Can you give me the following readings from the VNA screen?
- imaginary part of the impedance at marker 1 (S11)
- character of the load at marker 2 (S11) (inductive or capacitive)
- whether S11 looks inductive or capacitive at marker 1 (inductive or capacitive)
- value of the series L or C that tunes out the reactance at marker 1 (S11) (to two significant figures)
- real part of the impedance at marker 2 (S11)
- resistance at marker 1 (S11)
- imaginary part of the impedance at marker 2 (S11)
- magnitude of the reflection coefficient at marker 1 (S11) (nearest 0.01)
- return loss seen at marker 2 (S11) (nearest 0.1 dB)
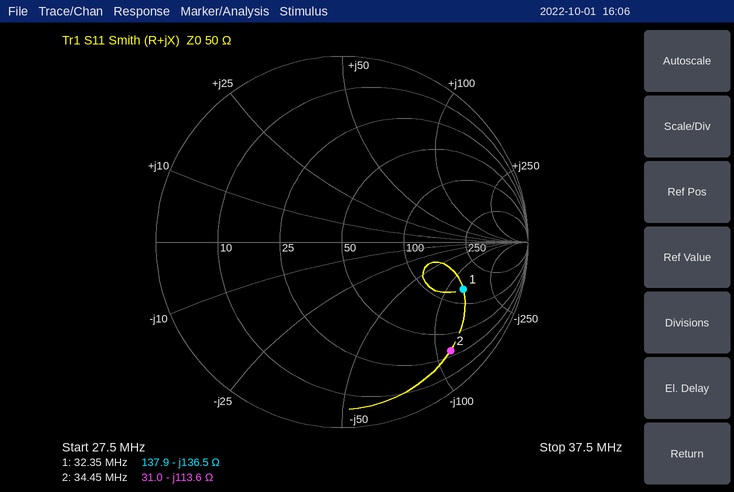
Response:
-136.5 Ω
capacitive
capacitive
670 nH
31.0 Ω
137.9 Ω
-113.6 Ω
0.70
1.7 dB
